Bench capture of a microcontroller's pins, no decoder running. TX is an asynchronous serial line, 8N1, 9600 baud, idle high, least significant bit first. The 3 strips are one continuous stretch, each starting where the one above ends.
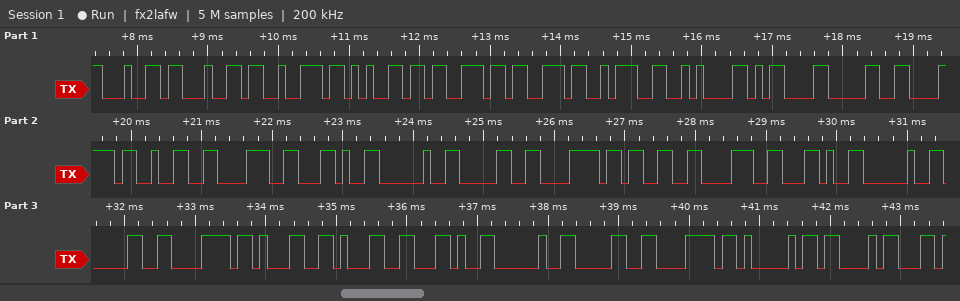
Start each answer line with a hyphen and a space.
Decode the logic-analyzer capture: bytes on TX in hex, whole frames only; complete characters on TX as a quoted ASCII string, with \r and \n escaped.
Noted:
- 64 64 72 65 73 73 3A 0A 0D 30 78 32 38 2C 20 30 78 33 38 2C 20 30 78 31 31 2C 20 30 78 41 43
- "ddress:\n\r0x28, 0x38, 0x11, 0xAC"
